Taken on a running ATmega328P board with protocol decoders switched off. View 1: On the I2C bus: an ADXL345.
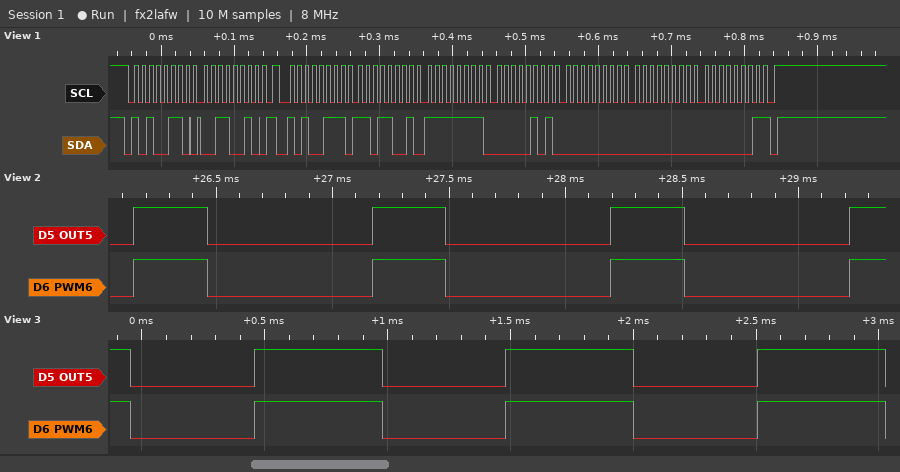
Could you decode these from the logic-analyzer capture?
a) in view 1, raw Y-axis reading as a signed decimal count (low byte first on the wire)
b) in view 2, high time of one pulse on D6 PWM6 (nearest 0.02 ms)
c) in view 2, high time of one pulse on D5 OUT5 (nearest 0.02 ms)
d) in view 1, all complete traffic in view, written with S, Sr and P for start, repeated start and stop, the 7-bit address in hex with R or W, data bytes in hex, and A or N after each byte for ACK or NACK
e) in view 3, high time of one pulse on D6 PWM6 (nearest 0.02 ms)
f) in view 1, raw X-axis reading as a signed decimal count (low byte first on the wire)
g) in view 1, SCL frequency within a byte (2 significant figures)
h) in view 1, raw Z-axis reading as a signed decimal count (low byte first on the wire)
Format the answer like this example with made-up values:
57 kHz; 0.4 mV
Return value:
5; 0.32 ms; 0.32 ms; S 53W A 32 A Sr 53R A D9 A FF A 05 A 00 A 00 A 01 N P; 0.52 ms; -39; 100 kHz; 256
